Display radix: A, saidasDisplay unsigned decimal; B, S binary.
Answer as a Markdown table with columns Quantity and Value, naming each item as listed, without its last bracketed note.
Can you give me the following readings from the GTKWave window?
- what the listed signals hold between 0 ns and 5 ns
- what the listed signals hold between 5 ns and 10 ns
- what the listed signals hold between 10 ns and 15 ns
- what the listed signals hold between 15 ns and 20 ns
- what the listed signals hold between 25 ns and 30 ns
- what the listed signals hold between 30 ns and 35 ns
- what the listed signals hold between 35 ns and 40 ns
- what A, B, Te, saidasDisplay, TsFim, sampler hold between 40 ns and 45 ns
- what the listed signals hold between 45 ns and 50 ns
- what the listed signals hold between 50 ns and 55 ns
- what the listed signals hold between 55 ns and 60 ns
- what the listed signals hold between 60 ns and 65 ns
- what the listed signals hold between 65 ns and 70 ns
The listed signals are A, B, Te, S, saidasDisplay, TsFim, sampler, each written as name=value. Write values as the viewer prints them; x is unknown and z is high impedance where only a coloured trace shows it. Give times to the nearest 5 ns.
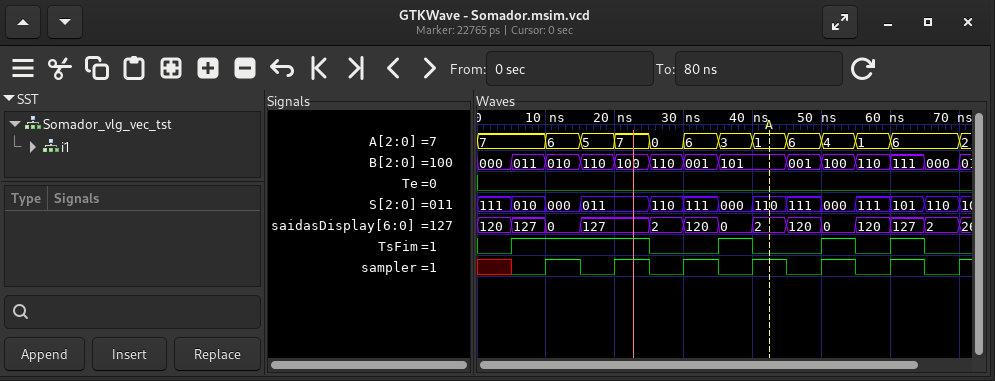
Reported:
| Quantity | Value |
|---|---|
| what the listed signals hold between 0 ns and 5 ns | A=7, B=000, Te=0, S=111, saidasDisplay=120, TsFim=0, sampler=x |
| what the listed signals hold between 5 ns and 10 ns | A=7, B=011, Te=0, S=010, saidasDisplay=127, TsFim=1, sampler=0 |
| what the listed signals hold between 10 ns and 15 ns | A=6, B=010, Te=0, S=000, saidasDisplay=0, TsFim=1, sampler=1 |
| what the listed signals hold between 15 ns and 20 ns | A=5, B=110, Te=0, S=011, saidasDisplay=127, TsFim=1, sampler=0 |
| what the listed signals hold between 25 ns and 30 ns | A=0, B=110, Te=0, S=110, saidasDisplay=2, TsFim=0, sampler=0 |
| what the listed signals hold between 30 ns and 35 ns | A=6, B=001, Te=0, S=111, saidasDisplay=120, TsFim=0, sampler=1 |
| what the listed signals hold between 35 ns and 40 ns | A=3, B=101, Te=0, S=000, saidasDisplay=0, TsFim=1, sampler=0 |
| what A, B, Te, saidasDisplay, TsFim, sampler hold between 40 ns and 45 ns | A=1, B=101, Te=0, saidasDisplay=2, TsFim=0, sampler=1 |
| what the listed signals hold between 45 ns and 50 ns | A=6, B=001, Te=0, S=111, saidasDisplay=120, TsFim=0, sampler=0 |
| what the listed signals hold between 50 ns and 55 ns | A=4, B=100, Te=0, S=000, saidasDisplay=0, TsFim=1, sampler=1 |
| what the listed signals hold between 55 ns and 60 ns | A=1, B=110, Te=0, S=111, saidasDisplay=120, TsFim=0, sampler=0 |
| what the listed signals hold between 60 ns and 65 ns | A=6, B=111, Te=0, S=101, saidasDisplay=127, TsFim=1, sampler=1 |
| what the listed signals hold between 65 ns and 70 ns | A=6, B=000, Te=0, S=110, saidasDisplay=2, TsFim=0, sampler=0 |
